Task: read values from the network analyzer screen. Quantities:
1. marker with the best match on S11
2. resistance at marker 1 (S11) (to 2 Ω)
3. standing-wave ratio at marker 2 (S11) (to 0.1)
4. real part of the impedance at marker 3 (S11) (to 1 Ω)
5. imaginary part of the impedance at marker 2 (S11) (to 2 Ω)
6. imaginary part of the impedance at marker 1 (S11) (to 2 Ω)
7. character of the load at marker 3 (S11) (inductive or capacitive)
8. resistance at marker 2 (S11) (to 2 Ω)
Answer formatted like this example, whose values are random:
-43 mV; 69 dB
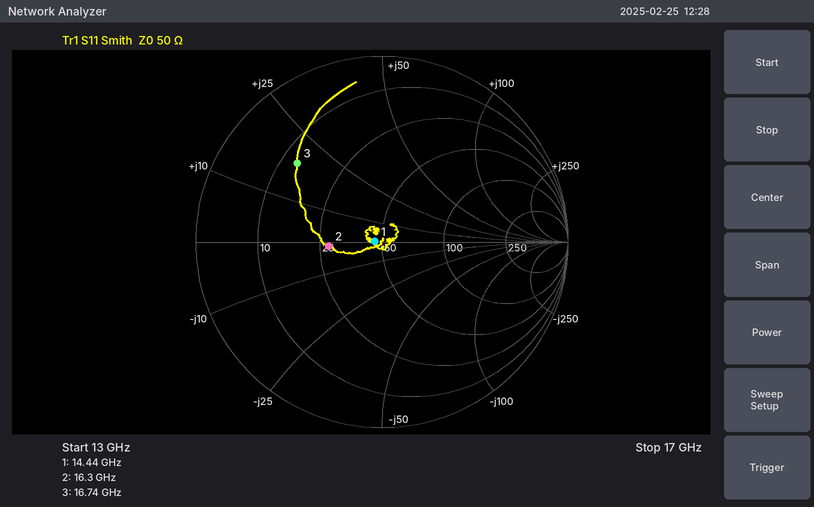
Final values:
marker 1; 46 Ω; 1.8; 13 Ω; -2 Ω; 0 Ω; inductive; 28 Ω
